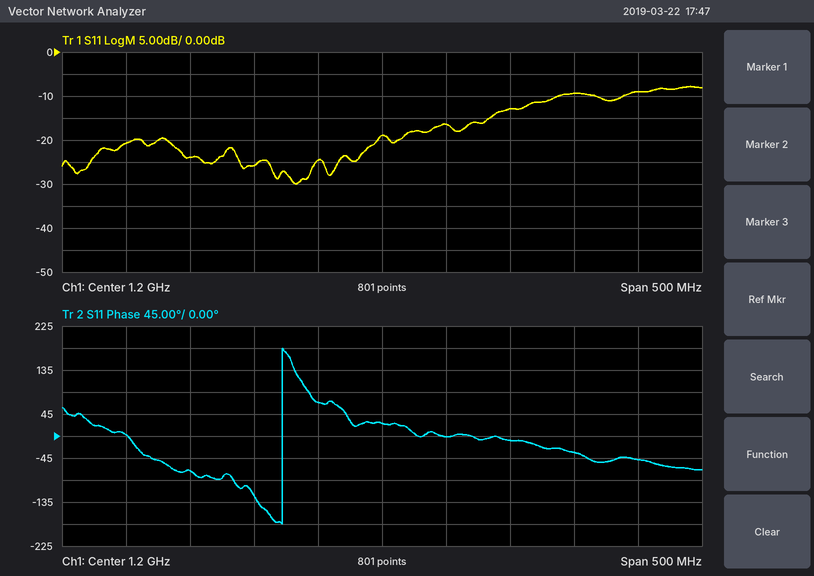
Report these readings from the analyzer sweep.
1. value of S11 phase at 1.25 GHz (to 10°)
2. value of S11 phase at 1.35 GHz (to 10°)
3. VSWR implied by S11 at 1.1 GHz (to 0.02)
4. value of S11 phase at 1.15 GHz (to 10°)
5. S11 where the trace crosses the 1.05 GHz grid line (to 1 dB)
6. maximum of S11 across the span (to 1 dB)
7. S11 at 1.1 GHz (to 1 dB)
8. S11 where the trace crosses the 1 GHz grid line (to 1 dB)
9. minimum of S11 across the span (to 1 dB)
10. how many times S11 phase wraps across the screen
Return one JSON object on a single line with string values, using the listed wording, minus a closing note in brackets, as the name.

{"value of S11 phase at 1.25 GHz": "0°", "value of S11 phase at 1.35 GHz": "-30°", "VSWR implied by S11 at 1.1 GHz": "1.10", "value of S11 phase at 1.15 GHz": "70°", "S11 where the trace crosses the 1.05 GHz grid line": "-24 dB", "maximum of S11 across the span": "-8 dB", "S11 at 1.1 GHz": "-26 dB", "S11 where the trace crosses the 1 GHz grid line": "-21 dB", "minimum of S11 across the span": "-30 dB", "how many times S11 phase wraps across the screen": "1"}
